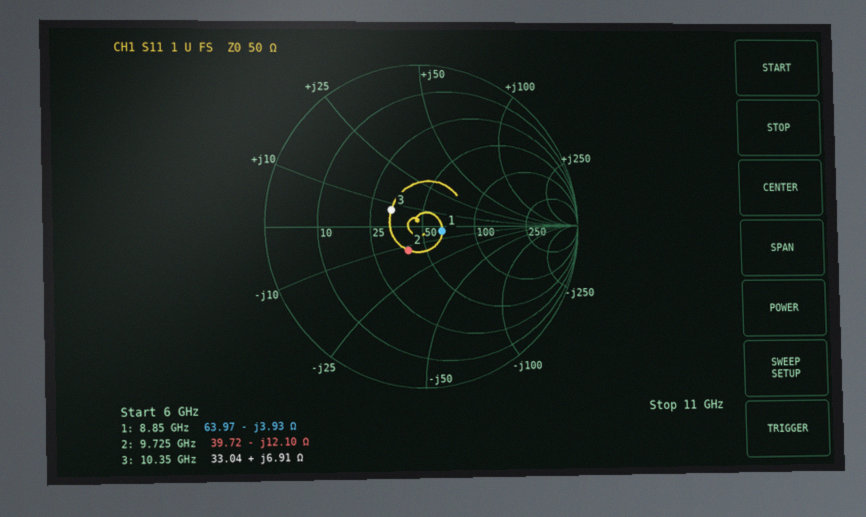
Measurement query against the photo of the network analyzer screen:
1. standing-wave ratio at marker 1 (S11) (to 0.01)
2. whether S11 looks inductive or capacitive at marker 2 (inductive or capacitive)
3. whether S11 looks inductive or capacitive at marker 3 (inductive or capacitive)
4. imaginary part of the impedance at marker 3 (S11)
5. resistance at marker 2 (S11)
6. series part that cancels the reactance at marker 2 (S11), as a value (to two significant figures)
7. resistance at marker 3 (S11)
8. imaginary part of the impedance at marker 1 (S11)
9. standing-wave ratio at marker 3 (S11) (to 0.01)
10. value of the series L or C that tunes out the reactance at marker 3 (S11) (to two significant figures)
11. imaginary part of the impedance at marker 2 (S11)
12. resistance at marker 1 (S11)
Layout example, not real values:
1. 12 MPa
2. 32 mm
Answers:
1. 1.29
2. capacitive
3. inductive
4. +6.91 Ω
5. 39.72 Ω
6. 200 pH
7. 33.04 Ω
8. -3.93 Ω
9. 1.56
10. 2.2 pF
11. -12.10 Ω
12. 63.97 Ω
